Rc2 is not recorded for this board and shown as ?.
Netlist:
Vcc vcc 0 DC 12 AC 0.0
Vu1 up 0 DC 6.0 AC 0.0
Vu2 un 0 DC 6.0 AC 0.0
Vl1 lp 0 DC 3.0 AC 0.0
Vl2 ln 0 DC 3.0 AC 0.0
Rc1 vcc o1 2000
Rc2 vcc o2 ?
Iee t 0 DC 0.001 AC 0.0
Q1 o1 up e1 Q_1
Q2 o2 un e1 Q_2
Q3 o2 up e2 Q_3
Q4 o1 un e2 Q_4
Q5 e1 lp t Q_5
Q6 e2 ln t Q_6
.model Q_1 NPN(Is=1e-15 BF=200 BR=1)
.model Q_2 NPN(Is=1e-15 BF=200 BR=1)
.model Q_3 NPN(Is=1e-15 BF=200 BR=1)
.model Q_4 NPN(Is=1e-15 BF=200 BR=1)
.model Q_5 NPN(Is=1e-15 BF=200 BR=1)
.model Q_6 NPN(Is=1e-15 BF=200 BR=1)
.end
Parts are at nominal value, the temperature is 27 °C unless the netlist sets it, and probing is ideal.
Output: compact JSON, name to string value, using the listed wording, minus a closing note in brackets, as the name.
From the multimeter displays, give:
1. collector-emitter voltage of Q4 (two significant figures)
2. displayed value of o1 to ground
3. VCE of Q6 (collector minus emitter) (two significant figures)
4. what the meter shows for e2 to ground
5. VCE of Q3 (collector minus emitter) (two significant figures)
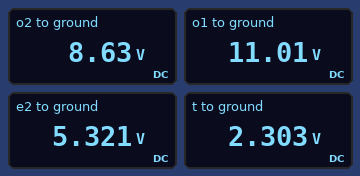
{"collector-emitter voltage of Q4": "5.7 V", "displayed value of o1 to ground": "11.01 V", "VCE of Q6 (collector minus emitter)": "3.0 V", "what the meter shows for e2 to ground": "5.321 V", "VCE of Q3 (collector minus emitter)": "3.3 V"}
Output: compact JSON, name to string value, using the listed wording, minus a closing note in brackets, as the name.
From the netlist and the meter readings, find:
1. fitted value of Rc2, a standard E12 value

{"fitted value of Rc2, a standard E12 value": "6.8 kΩ"}
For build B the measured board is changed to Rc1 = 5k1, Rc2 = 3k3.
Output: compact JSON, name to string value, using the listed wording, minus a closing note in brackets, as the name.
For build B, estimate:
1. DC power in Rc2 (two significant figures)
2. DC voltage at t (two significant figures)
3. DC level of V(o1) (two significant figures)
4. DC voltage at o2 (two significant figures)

{"DC power in Rc2": "810 µW", "DC voltage at t": "2.3 V", "DC level of V(o1)": "9.5 V", "DC voltage at o2": "10 V"}
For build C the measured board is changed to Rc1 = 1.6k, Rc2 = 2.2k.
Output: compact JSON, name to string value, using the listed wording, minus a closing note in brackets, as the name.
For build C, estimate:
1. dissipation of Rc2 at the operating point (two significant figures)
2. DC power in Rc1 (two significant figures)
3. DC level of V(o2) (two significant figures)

{"dissipation of Rc2 at the operating point": "540 µW", "DC power in Rc1": "390 µW", "DC level of V(o2)": "11 V"}
